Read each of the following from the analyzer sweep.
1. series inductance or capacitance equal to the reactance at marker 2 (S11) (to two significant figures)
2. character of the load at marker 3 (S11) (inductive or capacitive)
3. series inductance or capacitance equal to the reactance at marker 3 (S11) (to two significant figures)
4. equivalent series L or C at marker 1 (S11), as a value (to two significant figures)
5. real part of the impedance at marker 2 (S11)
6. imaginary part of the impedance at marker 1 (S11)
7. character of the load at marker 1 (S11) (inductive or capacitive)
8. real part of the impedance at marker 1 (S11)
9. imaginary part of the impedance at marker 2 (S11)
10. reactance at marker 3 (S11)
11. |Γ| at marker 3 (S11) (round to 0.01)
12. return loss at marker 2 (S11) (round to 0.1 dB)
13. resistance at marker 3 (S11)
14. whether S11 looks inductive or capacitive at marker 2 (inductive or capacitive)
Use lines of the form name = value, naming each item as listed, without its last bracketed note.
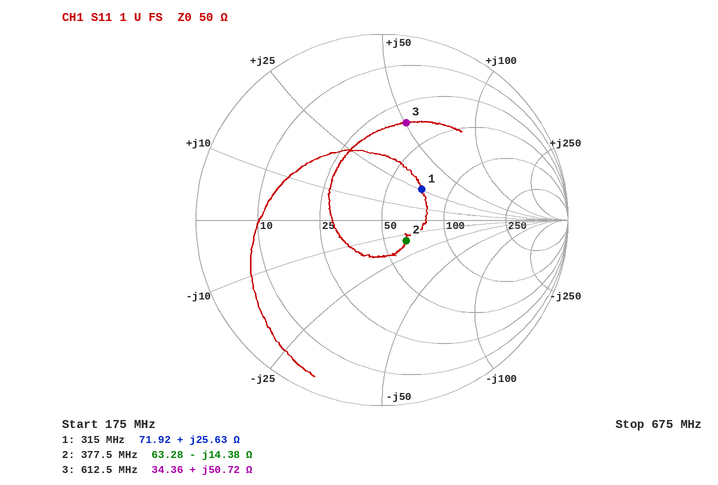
series inductance or capacitance equal to the reactance at marker 2 (S11) = 29 pF
character of the load at marker 3 (S11) = inductive
series inductance or capacitance equal to the reactance at marker 3 (S11) = 13 nH
equivalent series L or C at marker 1 (S11), as a value = 13 nH
real part of the impedance at marker 2 = 63.28 Ω
imaginary part of the impedance at marker 1 = +25.63 Ω
character of the load at marker 1 (S11) = inductive
real part of the impedance at marker 1 = 71.92 Ω
imaginary part of the impedance at marker 2 = -14.38 Ω
reactance at marker 3 = +50.72 Ω
|Γ| at marker 3 (S11) = 0.54
return loss at marker 2 (S11) = 15.3 dB
resistance at marker 3 = 34.36 Ω
whether S11 looks inductive or capacitive at marker 2 = capacitive
